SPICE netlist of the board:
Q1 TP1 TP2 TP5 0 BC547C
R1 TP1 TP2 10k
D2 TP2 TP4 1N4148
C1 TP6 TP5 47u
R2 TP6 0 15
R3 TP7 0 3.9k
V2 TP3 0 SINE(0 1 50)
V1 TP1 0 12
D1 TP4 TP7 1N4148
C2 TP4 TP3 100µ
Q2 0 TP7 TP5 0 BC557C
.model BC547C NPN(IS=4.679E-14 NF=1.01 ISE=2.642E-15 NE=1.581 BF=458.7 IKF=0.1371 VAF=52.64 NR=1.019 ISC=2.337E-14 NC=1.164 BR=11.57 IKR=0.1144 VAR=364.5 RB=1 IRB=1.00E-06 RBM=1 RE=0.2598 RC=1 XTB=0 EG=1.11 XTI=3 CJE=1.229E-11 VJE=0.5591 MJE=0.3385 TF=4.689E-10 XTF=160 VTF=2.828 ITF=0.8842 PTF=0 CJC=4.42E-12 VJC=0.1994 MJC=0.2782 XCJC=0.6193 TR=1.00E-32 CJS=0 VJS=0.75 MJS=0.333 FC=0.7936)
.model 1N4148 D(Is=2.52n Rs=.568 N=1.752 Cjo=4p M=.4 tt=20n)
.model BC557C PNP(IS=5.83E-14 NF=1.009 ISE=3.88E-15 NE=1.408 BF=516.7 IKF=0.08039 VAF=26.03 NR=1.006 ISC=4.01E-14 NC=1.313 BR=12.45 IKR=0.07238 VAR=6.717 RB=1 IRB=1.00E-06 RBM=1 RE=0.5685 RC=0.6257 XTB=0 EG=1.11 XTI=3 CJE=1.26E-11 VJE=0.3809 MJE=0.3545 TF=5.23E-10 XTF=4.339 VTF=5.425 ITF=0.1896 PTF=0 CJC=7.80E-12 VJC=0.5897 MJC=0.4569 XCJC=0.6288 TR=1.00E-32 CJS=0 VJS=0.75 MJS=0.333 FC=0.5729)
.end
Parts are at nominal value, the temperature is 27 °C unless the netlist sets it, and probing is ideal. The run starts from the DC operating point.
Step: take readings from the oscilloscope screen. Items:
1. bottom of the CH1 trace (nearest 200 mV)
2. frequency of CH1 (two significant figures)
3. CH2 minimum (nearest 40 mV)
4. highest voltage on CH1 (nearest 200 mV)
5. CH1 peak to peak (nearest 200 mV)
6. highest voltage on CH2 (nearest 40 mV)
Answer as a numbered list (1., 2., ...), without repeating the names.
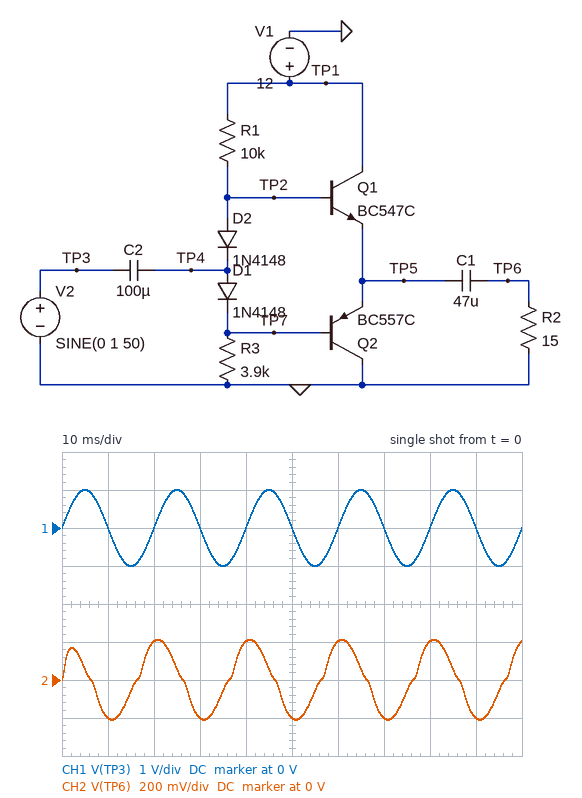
1. -1.0 V
2. 50 Hz
3. -200 mV
4. 1.0 V
5. 2.0 V
6. 200 mV
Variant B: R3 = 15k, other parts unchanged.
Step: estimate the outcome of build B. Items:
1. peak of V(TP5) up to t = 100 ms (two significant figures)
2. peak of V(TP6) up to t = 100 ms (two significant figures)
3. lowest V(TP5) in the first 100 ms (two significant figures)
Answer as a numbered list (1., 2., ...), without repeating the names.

1. 8.0 V
2. 210 mV
3. 6.2 V
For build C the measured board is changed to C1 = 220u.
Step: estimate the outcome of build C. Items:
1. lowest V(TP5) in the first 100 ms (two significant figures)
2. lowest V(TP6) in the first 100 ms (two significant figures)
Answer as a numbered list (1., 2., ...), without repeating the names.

1. 2.8 V
2. -630 mV
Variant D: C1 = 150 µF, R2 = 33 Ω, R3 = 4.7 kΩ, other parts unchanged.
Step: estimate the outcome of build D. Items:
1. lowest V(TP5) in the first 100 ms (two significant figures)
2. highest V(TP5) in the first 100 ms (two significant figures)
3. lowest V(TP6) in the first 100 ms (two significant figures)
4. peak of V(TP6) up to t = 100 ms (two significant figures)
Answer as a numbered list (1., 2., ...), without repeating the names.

1. 3.2 V
2. 4.9 V
3. -760 mV
4. 730 mV
